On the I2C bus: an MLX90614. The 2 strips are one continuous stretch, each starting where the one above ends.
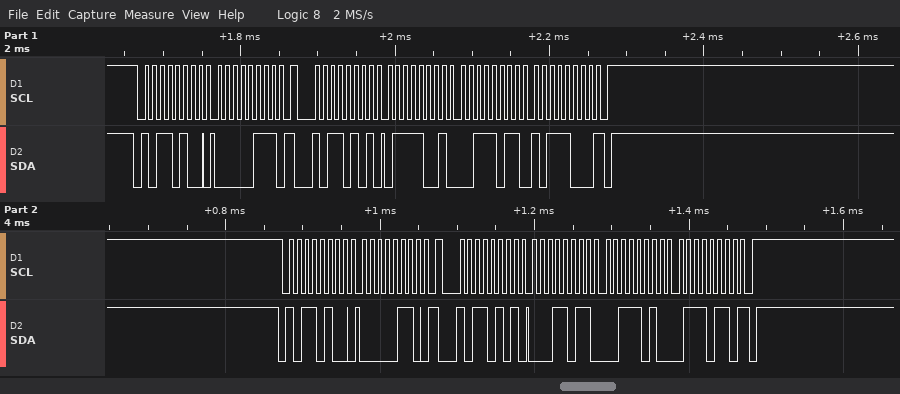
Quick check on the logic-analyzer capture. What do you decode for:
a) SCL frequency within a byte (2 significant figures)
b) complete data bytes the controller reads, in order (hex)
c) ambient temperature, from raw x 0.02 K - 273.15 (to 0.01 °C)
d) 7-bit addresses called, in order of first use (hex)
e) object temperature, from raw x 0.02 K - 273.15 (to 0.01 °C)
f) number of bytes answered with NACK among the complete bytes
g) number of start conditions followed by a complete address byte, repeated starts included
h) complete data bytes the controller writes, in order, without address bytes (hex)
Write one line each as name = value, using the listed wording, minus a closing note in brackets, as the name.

SCL frequency within a byte = 100 kHz
complete data bytes the controller reads, in order = 79 3B B8 1B 3A 76
ambient temperature, from raw x 0.02 K - 273.15 = 24.35 °C
7-bit addresses called, in order of first use = 0x5A
object temperature, from raw x 0.02 K - 273.15 = 31.35 °C
number of bytes answered with NACK among the complete bytes = 2
number of start conditions followed by a complete address byte, repeated starts included = 4
complete data bytes the controller writes, in order, without address bytes = 07 06
